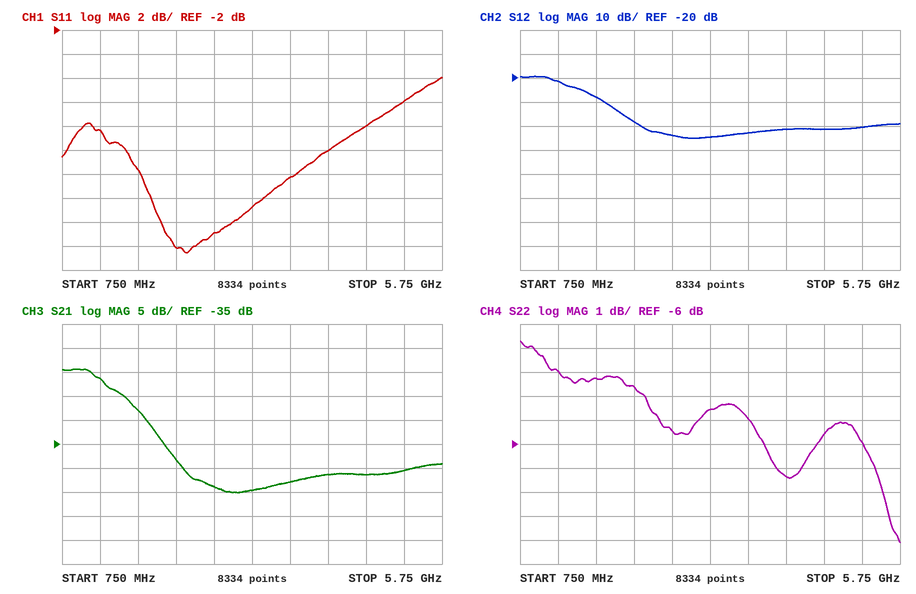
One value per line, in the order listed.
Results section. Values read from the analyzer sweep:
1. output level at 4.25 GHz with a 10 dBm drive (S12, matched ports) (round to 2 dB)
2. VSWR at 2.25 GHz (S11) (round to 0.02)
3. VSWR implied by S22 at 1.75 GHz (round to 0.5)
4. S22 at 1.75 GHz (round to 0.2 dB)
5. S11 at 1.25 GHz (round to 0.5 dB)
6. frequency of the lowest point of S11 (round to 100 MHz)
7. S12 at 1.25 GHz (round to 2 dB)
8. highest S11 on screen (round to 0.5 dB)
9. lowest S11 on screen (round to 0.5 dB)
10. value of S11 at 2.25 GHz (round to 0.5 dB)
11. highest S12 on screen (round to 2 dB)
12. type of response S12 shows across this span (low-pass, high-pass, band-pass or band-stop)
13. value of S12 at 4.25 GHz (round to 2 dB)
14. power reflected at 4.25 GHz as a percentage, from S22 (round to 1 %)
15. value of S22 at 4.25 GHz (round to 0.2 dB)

-32 dBm
1.22
5.5
-3.2 dB
-10.5 dB
2.4 GHz
-22 dB
-6.0 dB
-20.5 dB
-20.0 dB
-20 dB
low-pass
-42 dB
18 %
-7.4 dB
